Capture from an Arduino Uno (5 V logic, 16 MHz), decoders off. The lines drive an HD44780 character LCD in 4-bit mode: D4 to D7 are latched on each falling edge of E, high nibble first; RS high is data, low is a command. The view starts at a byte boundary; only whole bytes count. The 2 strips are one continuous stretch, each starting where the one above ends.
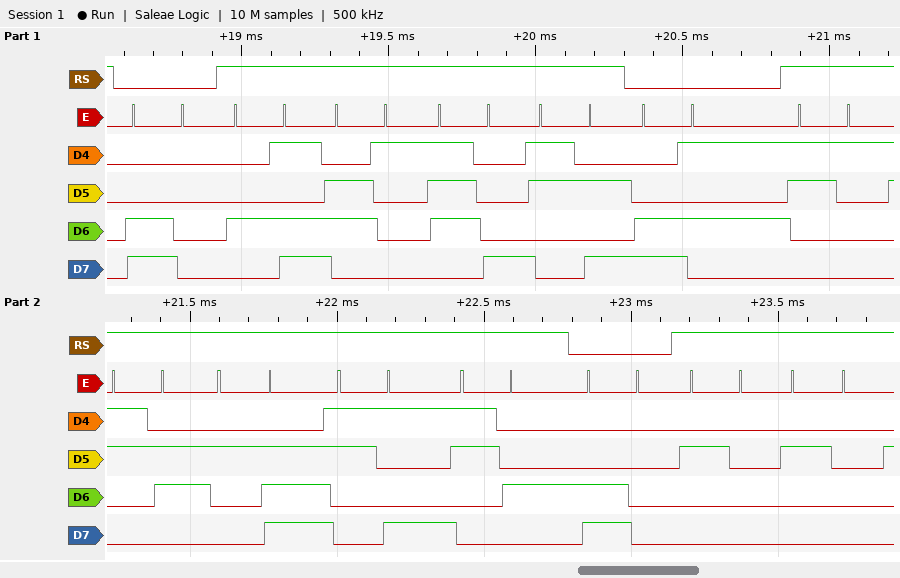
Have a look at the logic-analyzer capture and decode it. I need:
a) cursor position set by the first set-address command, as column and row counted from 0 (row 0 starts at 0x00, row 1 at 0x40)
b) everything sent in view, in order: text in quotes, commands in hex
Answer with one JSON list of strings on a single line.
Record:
["column 0, row 1", "0xC0 \"Max:\" 0xC5 \"16.94\" 0xC0 \"  \""]
